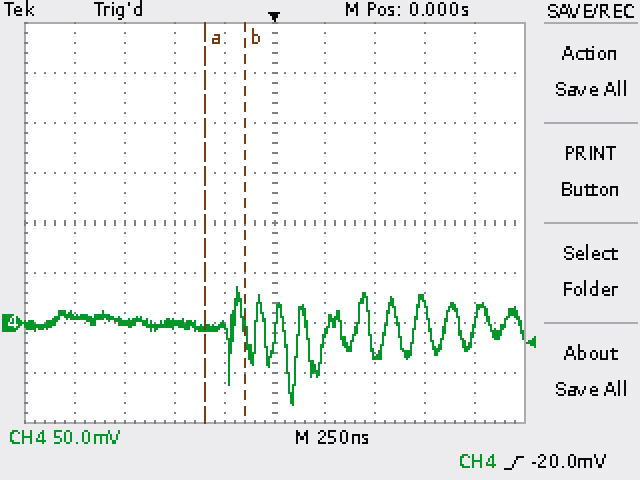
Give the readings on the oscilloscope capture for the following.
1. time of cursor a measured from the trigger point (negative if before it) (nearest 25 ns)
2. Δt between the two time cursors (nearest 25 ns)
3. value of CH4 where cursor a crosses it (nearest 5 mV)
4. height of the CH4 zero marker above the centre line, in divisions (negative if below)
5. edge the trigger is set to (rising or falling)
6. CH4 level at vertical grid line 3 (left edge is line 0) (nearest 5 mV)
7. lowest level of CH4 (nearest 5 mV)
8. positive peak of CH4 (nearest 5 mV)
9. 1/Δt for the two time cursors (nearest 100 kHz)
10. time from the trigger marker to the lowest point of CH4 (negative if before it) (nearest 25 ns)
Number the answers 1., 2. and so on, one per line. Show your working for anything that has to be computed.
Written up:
1. -350 ns
2. 200 ns
3. -5 mV
4. -2.0 div
5. rising
6. 0 mV
7. -80 mV
8. 35 mV
9. 1 / 200 ns ≈ 5.0 MHz
10. +100 ns
